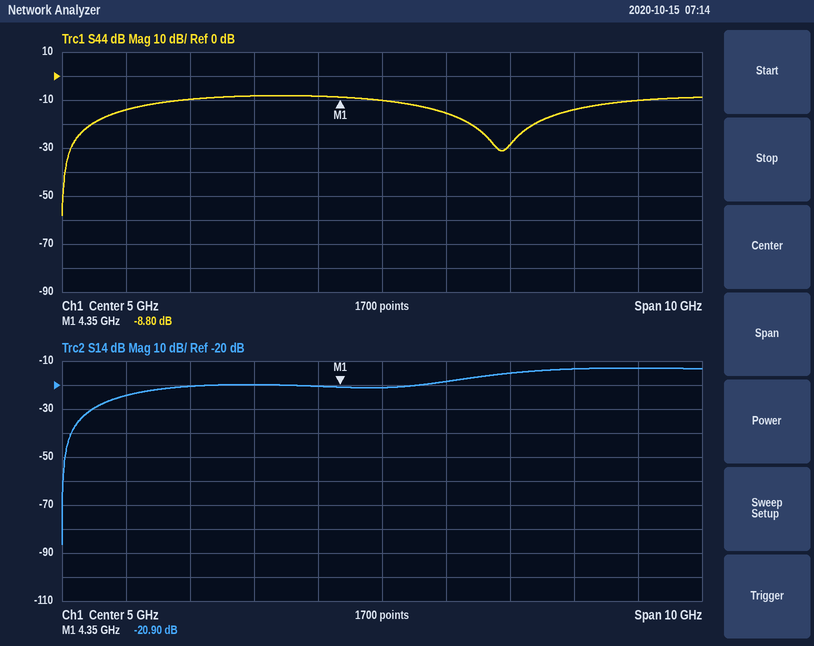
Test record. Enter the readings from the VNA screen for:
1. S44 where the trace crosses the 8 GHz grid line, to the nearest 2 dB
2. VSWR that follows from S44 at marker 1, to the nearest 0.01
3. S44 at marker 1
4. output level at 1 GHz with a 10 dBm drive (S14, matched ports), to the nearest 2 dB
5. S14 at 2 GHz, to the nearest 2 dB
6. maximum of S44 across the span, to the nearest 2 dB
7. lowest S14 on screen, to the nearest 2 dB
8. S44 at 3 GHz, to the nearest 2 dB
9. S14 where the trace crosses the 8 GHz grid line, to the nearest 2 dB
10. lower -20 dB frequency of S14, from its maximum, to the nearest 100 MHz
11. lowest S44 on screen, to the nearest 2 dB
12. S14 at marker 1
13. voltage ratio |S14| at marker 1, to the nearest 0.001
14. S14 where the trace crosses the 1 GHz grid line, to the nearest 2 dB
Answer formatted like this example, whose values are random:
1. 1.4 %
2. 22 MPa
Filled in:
1. -14 dB
2. 2.14
3. -8.80 dB
4. -14 dBm
5. -20 dB
6. -8 dB
7. -86 dB
8. -8 dB
9. -14 dB
10. 300 MHz
11. -58 dB
12. -20.90 dB
13. 0.090
14. -24 dB
